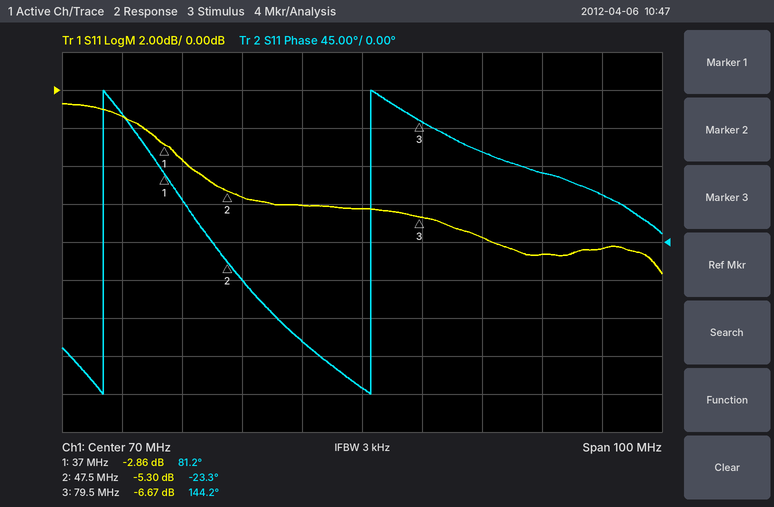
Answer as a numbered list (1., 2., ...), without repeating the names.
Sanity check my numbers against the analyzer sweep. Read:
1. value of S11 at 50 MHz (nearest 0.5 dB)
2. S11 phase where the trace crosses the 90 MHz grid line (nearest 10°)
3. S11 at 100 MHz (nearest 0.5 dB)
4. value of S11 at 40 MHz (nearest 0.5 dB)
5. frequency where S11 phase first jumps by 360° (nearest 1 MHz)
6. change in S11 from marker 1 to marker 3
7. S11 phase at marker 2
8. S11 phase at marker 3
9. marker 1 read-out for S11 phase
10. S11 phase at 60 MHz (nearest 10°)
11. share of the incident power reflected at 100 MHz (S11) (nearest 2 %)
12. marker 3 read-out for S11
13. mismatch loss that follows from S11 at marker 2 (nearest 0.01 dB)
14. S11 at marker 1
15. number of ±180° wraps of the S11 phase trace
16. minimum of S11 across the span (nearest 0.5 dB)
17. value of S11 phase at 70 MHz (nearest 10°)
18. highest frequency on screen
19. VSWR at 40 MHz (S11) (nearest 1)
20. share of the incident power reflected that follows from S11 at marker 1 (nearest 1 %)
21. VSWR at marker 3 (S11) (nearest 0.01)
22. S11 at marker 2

1. -5.5 dB
2. 110°
3. -8.5 dB
4. -3.5 dB
5. 27 MHz
6. -3.81 dB
7. -23.3°
8. 144.2°
9. 81.2°
10. -120°
11. 14 %
12. -6.67 dB
13. 1.52 dB
14. -2.86 dB
15. 2
16. -9.5 dB
17. -170°
18. 120 MHz
19. 5
20. 52 %
21. 2.73
22. -5.30 dB
